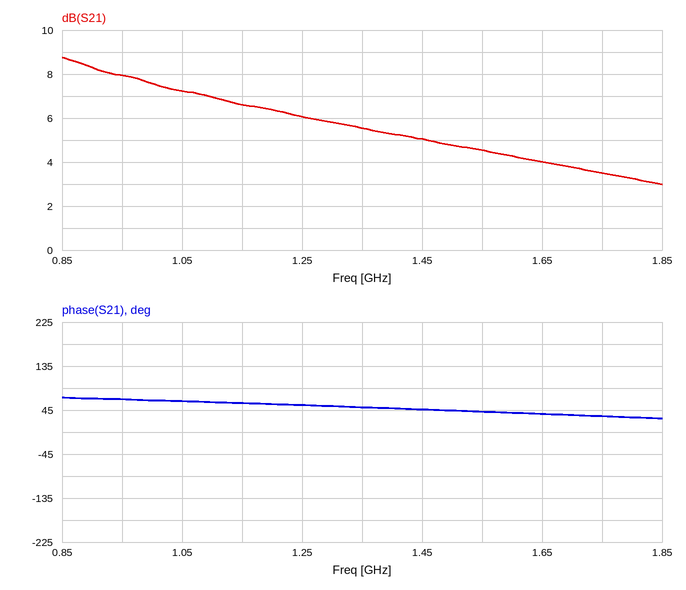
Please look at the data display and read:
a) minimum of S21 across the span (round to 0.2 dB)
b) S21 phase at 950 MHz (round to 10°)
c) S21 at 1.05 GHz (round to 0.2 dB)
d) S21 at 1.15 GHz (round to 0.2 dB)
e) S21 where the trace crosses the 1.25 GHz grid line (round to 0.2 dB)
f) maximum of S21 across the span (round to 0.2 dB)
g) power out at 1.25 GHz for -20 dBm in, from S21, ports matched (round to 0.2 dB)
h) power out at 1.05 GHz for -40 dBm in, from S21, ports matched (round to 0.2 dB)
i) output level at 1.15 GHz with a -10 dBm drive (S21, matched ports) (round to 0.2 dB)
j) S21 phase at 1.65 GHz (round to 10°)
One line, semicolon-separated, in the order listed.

3.0 dB; 70°; 7.2 dB; 6.6 dB; 6.0 dB; 8.8 dB; -14.0 dBm; -32.8 dBm; -3.4 dBm; 40°
